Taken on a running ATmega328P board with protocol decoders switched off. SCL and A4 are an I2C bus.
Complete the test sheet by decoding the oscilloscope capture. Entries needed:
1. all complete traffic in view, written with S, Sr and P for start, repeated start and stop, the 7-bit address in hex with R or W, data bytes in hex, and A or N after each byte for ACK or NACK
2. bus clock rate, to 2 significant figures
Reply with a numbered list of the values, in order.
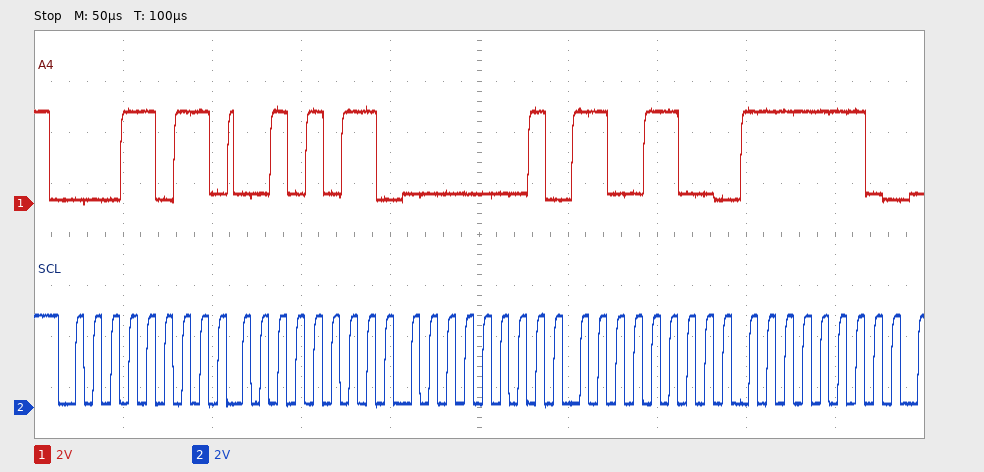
1. S 0DR A 2B A 01 A CC A FE A
2. 100 kHz
